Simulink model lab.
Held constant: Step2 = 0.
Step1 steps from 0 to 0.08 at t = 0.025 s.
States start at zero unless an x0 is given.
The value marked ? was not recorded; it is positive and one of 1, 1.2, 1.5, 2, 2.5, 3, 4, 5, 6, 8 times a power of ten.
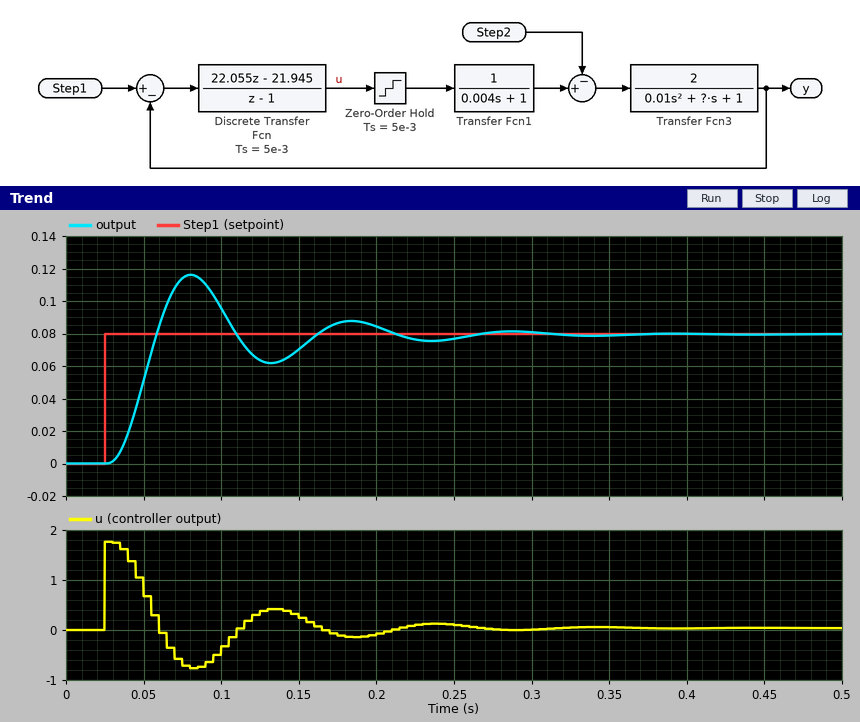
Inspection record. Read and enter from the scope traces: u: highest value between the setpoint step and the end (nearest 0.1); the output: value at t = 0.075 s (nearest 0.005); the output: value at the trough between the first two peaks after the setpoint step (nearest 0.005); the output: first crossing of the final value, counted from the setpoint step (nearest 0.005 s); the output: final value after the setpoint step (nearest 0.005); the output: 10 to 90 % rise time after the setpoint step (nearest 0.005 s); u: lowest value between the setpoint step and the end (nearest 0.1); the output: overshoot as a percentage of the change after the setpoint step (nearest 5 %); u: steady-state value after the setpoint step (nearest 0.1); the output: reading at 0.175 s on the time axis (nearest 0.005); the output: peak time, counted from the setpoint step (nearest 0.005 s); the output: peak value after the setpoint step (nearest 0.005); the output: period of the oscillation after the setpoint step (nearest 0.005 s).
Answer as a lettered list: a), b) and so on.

a) 1.8
b) 0.115
c) 0.060
d) 0.035 s
e) 0.080
f) 0.020 s
g) -0.8
h) 45 %
i) 0.0
j) 0.085
k) 0.055 s
l) 0.115
m) 0.105 s
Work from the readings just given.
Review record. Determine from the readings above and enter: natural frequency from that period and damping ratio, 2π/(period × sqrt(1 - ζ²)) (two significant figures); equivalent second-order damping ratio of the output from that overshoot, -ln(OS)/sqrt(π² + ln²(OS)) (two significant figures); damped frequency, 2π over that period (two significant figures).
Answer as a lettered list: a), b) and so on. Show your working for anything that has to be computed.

a) 2π / (0.105 × sqrt(1 - 0.25²)) = 62 rad/s
b) ln(0.45) = -0.799; 0.799 / sqrt(9.870 + 0.638) = 0.25
c) 2π / 0.105 = 60 rad/s
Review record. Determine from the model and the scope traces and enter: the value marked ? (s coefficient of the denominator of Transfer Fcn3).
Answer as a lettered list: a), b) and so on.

a) 0.6
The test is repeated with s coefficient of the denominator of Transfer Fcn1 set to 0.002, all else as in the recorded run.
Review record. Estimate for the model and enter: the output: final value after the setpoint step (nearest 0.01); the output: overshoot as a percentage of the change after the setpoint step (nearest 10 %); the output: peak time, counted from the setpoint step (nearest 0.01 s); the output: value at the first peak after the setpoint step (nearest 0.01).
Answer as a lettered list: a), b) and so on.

a) 0.08
b) 40 %
c) 0.05 s
d) 0.11
